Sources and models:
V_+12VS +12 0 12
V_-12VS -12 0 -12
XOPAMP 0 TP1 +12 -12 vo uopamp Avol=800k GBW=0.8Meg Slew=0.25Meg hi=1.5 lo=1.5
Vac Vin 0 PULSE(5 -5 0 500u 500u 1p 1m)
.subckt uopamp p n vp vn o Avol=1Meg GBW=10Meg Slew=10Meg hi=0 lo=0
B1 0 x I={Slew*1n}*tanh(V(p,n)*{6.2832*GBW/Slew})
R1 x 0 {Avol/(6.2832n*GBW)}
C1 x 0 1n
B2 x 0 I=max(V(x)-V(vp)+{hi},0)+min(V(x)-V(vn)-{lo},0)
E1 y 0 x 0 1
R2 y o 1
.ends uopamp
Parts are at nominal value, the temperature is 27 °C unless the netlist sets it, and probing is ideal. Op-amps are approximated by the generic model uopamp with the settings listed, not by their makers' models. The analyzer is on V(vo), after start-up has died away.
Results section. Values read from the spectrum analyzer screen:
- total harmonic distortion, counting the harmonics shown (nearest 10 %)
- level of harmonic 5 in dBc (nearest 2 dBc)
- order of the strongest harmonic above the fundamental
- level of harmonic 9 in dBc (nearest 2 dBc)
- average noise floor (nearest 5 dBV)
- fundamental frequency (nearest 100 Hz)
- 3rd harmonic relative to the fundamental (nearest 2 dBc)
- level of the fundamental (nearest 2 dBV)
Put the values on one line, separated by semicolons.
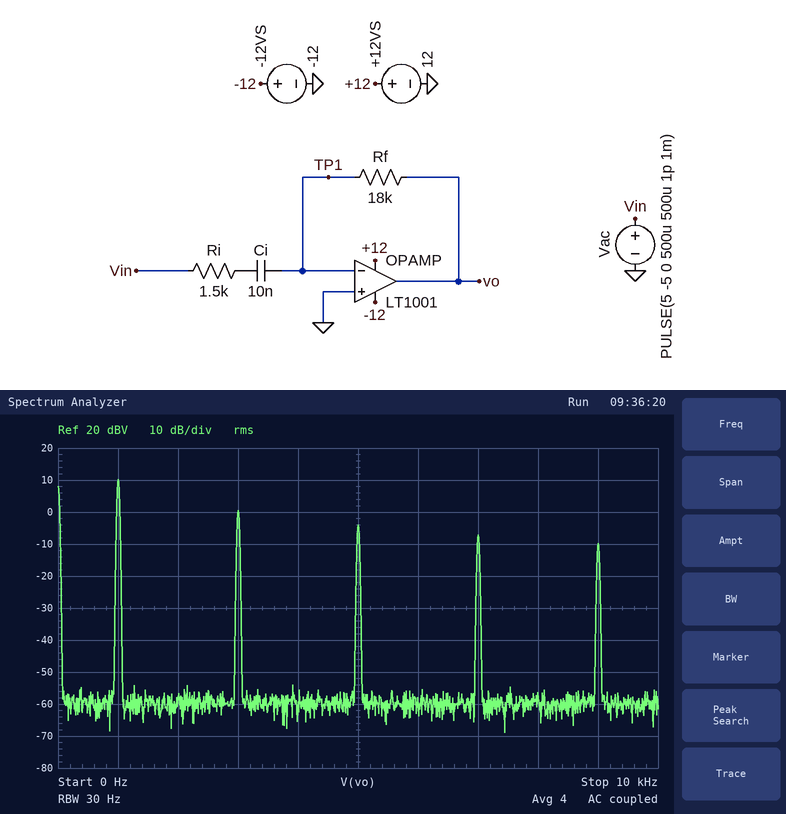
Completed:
40 %; -14 dBc; 3; -20 dBc; -60 dBV; 1.0 kHz; -10 dBc; 10 dBV
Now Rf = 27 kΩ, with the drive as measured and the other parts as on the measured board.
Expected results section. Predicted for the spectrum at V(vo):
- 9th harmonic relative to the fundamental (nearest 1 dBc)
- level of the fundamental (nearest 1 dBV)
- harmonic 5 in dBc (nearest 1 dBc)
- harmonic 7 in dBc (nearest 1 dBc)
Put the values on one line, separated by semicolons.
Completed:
-19 dBc; 14 dBV; -13 dBc; -16 dBc
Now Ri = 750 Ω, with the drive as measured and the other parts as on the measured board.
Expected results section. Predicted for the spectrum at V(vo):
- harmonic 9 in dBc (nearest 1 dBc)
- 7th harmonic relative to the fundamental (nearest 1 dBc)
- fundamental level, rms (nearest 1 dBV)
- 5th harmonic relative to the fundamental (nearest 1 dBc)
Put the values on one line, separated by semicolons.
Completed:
-17 dBc; -15 dBc; 10 dBV; -13 dBc
